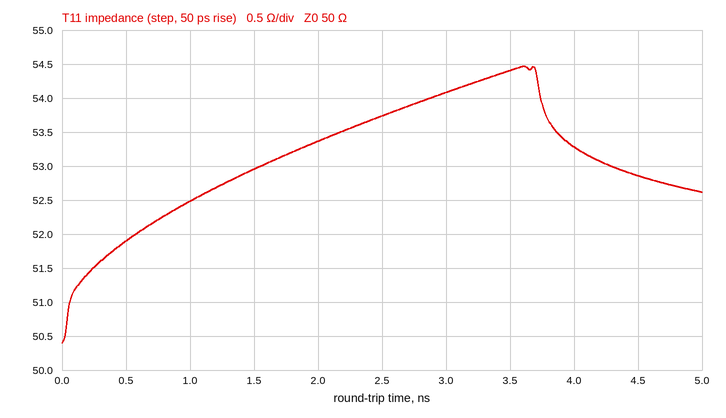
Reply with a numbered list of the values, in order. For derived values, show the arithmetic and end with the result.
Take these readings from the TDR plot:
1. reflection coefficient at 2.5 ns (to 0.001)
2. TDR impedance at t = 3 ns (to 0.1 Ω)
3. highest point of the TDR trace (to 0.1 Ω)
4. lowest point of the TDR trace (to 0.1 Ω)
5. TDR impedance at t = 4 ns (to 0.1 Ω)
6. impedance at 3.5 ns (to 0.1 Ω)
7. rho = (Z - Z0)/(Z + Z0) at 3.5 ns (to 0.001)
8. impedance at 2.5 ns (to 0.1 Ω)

1. (53.7 − 50)/(53.7 + 50) ≈ +0.036
2. 54.1 Ω
3. 54.5 Ω
4. 50.4 Ω
5. 53.3 Ω
6. 54.4 Ω
7. (54.4 − 50)/(54.4 + 50) ≈ +0.042
8. 53.7 Ω
